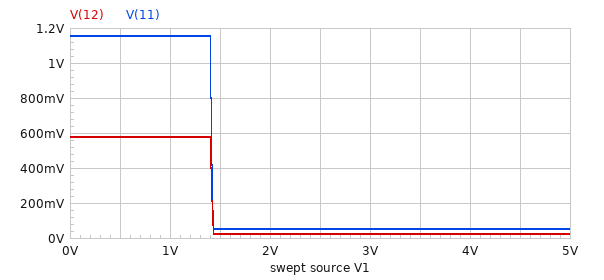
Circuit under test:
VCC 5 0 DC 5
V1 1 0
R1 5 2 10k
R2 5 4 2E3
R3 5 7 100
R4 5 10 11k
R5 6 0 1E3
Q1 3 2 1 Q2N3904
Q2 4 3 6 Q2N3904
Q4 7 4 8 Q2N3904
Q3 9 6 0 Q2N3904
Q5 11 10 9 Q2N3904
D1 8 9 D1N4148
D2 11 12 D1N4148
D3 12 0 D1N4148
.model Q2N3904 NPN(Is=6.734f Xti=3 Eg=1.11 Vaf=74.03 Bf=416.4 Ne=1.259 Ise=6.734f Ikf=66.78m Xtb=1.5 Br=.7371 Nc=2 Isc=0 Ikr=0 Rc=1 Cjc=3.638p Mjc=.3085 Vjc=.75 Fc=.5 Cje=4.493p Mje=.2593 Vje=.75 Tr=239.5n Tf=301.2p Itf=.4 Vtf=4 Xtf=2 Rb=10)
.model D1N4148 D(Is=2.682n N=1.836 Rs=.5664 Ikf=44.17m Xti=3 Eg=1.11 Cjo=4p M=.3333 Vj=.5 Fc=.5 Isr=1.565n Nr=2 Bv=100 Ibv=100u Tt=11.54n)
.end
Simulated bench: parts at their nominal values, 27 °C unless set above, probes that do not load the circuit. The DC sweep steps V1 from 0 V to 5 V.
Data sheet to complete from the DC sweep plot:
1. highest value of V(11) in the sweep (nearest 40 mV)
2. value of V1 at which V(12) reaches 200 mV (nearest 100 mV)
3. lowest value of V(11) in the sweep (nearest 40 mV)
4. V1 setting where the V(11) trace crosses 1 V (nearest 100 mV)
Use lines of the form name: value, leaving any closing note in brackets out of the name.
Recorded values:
highest value of V(11) in the sweep: 1.16 V
value of V1 at which V(12) reaches 200 mV: 1.4 V
lowest value of V(11) in the sweep: 40 mV
V1 setting where the V(11) trace crosses 1 V: 1.4 V
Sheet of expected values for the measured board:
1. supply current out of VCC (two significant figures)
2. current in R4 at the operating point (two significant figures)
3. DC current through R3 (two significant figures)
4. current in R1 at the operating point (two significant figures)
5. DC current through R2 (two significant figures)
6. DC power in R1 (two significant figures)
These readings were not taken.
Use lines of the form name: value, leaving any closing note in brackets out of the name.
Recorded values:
supply current out of VCC: 940 µA
current in R4 at the operating point: 290 µA
DC current through R3: 210 µA
current in R1 at the operating point: 430 µA
DC current through R2: 2.0 µA
DC power in R1: 1.9 mW
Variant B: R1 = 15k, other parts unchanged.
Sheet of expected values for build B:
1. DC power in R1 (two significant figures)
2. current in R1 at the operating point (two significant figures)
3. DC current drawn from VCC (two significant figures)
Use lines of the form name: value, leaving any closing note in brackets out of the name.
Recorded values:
DC power in R1: 1.3 mW
current in R1 at the operating point: 290 µA
DC current drawn from VCC: 800 µA
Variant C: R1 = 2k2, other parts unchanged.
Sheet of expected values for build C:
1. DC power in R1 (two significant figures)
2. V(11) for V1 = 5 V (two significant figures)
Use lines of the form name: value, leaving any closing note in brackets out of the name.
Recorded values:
DC power in R1: 8.3 mW
V(11) for V1 = 5 V: 48 mV
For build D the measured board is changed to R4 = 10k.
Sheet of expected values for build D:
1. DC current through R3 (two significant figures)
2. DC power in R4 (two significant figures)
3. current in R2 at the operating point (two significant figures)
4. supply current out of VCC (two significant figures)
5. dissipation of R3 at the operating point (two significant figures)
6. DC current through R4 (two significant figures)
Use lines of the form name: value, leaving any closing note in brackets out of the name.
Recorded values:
DC current through R3: 230 µA
DC power in R4: 1.0 mW
current in R2 at the operating point: 2.1 µA
supply current out of VCC: 990 µA
dissipation of R3 at the operating point: 5.4 µW
DC current through R4: 320 µA
